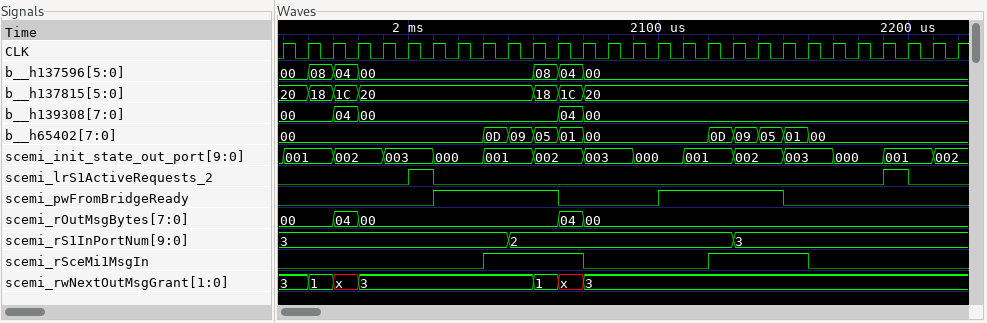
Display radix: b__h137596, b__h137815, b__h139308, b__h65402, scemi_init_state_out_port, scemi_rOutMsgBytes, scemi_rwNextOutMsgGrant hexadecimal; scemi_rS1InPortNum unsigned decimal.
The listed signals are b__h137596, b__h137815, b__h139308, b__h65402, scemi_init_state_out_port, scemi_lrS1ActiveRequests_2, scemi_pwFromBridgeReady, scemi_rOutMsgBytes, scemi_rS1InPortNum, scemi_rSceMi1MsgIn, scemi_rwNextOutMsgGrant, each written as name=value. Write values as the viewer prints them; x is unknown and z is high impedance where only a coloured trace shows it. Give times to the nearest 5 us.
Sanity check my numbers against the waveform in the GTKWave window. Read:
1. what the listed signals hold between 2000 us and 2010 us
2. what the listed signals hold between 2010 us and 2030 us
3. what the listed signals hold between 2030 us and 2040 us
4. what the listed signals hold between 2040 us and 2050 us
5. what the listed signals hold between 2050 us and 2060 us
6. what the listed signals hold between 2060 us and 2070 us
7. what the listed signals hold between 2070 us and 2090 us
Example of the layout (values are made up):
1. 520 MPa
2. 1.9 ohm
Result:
1. b__h137596=00, b__h137815=20, b__h139308=00, b__h65402=00, scemi_init_state_out_port=003, scemi_lrS1ActiveRequests_2=1, scemi_pwFromBridgeReady=0, scemi_rOutMsgBytes=00, scemi_rS1InPortNum=3, scemi_rSceMi1MsgIn=0, scemi_rwNextOutMsgGrant=3
2. b__h137596=00, b__h137815=20, b__h139308=00, b__h65402=00, scemi_init_state_out_port=000, scemi_lrS1ActiveRequests_2=0, scemi_pwFromBridgeReady=1, scemi_rOutMsgBytes=00, scemi_rS1InPortNum=3, scemi_rSceMi1MsgIn=0, scemi_rwNextOutMsgGrant=3
3. b__h137596=00, b__h137815=20, b__h139308=00, b__h65402=0D, scemi_init_state_out_port=001, scemi_lrS1ActiveRequests_2=0, scemi_pwFromBridgeReady=1, scemi_rOutMsgBytes=00, scemi_rS1InPortNum=3, scemi_rSceMi1MsgIn=1, scemi_rwNextOutMsgGrant=3
4. b__h137596=00, b__h137815=20, b__h139308=00, b__h65402=09, scemi_init_state_out_port=001, scemi_lrS1ActiveRequests_2=0, scemi_pwFromBridgeReady=1, scemi_rOutMsgBytes=00, scemi_rS1InPortNum=2, scemi_rSceMi1MsgIn=1, scemi_rwNextOutMsgGrant=3
5. b__h137596=08, b__h137815=18, b__h139308=00, b__h65402=05, scemi_init_state_out_port=002, scemi_lrS1ActiveRequests_2=0, scemi_pwFromBridgeReady=1, scemi_rOutMsgBytes=00, scemi_rS1InPortNum=2, scemi_rSceMi1MsgIn=1, scemi_rwNextOutMsgGrant=1
6. b__h137596=04, b__h137815=1C, b__h139308=04, b__h65402=01, scemi_init_state_out_port=002, scemi_lrS1ActiveRequests_2=0, scemi_pwFromBridgeReady=0, scemi_rOutMsgBytes=04, scemi_rS1InPortNum=2, scemi_rSceMi1MsgIn=1, scemi_rwNextOutMsgGrant=x
7. b__h137596=00, b__h137815=20, b__h139308=00, b__h65402=00, scemi_init_state_out_port=003, scemi_lrS1ActiveRequests_2=0, scemi_pwFromBridgeReady=0, scemi_rOutMsgBytes=00, scemi_rS1InPortNum=2, scemi_rSceMi1MsgIn=0, scemi_rwNextOutMsgGrant=3
